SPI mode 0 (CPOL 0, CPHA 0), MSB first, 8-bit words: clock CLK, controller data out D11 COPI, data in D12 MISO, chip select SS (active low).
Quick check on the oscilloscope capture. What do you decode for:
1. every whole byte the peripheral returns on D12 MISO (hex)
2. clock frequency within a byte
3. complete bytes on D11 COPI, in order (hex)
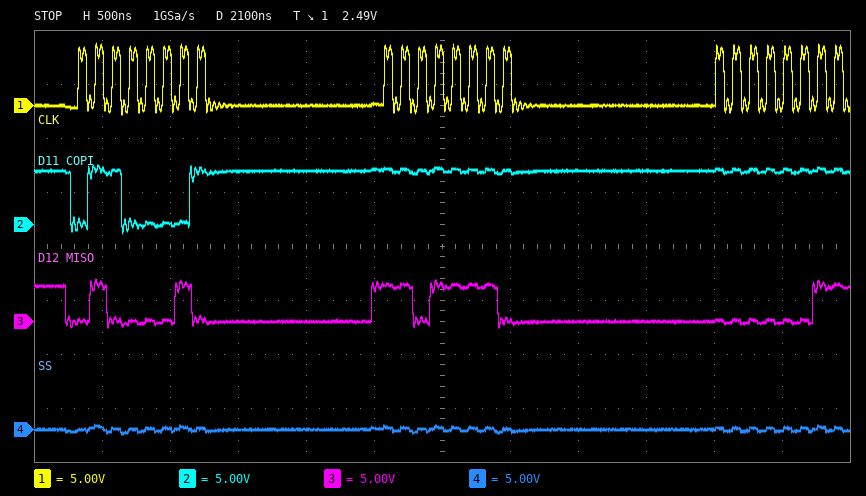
42 DE 03
8 MHz
61 FF FF
